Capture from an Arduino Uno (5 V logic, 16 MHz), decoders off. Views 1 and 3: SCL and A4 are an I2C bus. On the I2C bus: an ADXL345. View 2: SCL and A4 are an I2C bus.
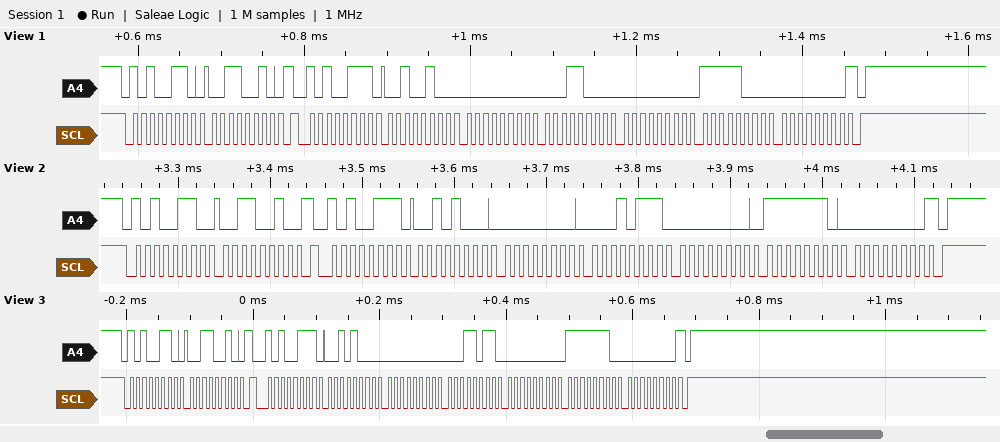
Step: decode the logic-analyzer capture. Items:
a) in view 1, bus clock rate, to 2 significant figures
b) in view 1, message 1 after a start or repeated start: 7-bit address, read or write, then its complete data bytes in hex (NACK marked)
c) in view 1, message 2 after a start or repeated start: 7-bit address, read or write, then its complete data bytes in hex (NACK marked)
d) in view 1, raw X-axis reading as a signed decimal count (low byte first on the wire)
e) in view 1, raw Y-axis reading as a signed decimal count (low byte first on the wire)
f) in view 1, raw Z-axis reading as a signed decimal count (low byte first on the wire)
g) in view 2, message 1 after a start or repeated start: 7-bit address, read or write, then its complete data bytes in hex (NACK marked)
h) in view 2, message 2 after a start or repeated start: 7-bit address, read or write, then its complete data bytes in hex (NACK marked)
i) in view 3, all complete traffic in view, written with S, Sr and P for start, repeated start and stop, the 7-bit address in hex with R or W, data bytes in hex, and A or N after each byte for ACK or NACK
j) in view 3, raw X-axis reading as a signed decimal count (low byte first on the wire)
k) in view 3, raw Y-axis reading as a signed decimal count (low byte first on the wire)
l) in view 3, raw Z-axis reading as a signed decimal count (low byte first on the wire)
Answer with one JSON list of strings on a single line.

["100 kHz", "0x53 write: 32", "0x53 read: 24 00 18 00 F8 00 NACK", "36", "24", "248", "0x53 write: 32", "0x53 read: 28 00 17 00 FE 00 NACK", "S 53W A 32 A Sr 53R A 28 A 00 A 1B A 00 A FE A 00 N P", "40", "27", "254"]
